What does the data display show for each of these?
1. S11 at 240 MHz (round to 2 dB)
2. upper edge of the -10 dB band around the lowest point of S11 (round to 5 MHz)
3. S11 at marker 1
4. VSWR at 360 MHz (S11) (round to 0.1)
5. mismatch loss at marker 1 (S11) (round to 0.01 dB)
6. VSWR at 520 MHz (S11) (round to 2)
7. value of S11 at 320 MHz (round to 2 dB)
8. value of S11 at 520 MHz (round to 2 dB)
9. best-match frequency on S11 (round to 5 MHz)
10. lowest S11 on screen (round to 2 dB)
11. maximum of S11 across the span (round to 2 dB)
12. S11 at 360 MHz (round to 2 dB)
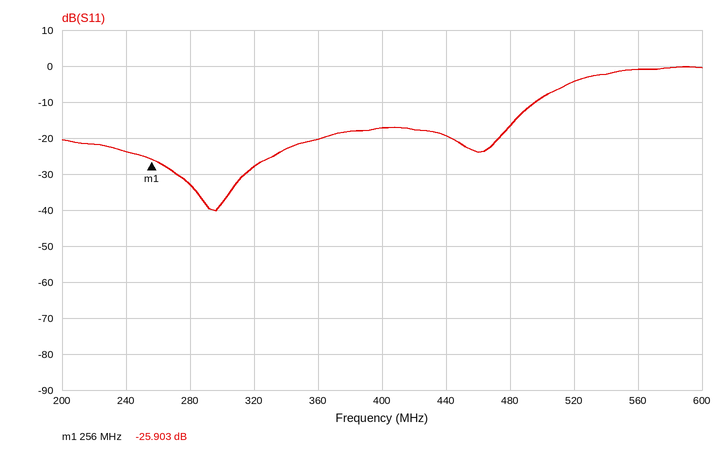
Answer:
-24 dB
495 MHz
-25.903 dB
1.2
0.01 dB
4
-28 dB
-4 dB
295 MHz
-40 dB
0 dB
-20 dB
